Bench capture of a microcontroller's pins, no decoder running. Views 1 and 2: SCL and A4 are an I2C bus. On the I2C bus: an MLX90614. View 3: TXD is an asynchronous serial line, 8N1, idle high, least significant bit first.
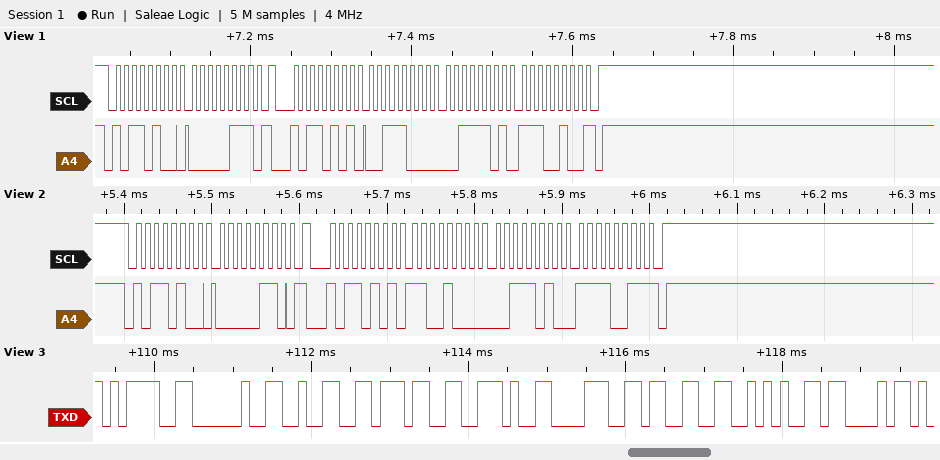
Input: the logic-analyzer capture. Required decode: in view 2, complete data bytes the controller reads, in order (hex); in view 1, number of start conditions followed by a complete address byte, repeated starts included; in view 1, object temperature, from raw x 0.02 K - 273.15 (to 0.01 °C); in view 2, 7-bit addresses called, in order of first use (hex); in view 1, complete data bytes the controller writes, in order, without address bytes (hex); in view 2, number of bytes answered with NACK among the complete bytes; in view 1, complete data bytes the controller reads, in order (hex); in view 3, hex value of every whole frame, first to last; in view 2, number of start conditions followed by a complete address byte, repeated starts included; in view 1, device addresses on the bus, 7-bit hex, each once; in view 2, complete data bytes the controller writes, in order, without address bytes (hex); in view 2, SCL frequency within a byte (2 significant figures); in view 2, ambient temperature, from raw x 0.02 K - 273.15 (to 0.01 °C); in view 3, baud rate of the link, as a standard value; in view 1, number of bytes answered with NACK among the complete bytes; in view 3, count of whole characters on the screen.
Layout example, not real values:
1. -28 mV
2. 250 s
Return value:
1. C8 3A F3
2. 2
3. 40.29 °C
4. 0x5A
5. 07
6. 1
7. 38 3D E4
8. 3D 20 32 37 2E 38 33 2A 43
9. 2
10. 0x5A
11. 06
12. 100 kHz
13. 27.81 °C
14. 9600 baud
15. 1
16. 9
